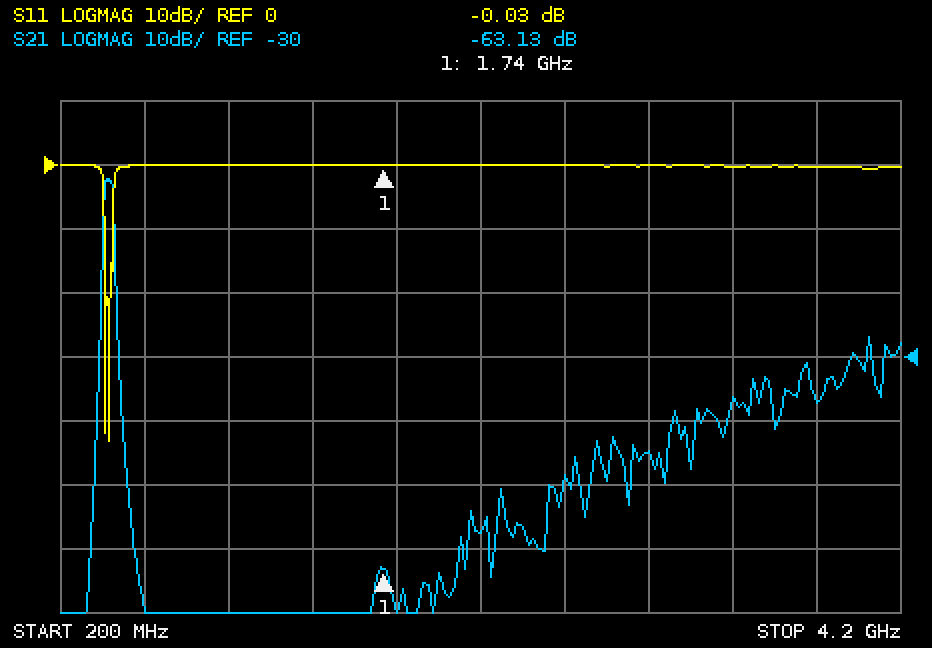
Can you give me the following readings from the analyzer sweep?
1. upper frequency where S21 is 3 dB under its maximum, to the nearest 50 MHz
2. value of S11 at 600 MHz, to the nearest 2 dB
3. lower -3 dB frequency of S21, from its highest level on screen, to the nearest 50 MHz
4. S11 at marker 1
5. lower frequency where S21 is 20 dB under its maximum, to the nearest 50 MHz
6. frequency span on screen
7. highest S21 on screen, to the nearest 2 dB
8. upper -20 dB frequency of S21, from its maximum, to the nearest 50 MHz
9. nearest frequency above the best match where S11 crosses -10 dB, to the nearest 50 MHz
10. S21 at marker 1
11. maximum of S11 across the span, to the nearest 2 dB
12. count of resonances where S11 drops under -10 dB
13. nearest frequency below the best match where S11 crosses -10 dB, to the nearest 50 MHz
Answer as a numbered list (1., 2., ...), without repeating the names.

1. 450 MHz
2. 0 dB
3. 400 MHz
4. -0.03 dB
5. 400 MHz
6. 4 GHz
7. -2 dB
8. 450 MHz
9. 450 MHz
10. -63.13 dB
11. 0 dB
12. 2
13. 400 MHz
